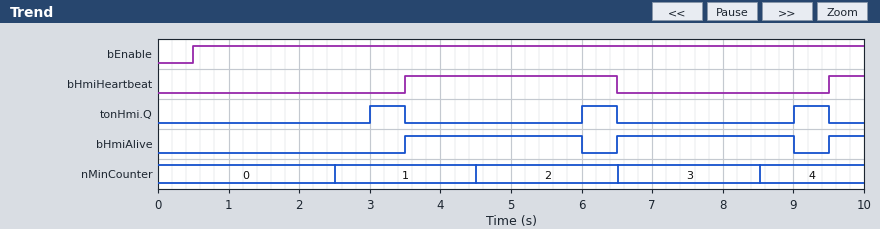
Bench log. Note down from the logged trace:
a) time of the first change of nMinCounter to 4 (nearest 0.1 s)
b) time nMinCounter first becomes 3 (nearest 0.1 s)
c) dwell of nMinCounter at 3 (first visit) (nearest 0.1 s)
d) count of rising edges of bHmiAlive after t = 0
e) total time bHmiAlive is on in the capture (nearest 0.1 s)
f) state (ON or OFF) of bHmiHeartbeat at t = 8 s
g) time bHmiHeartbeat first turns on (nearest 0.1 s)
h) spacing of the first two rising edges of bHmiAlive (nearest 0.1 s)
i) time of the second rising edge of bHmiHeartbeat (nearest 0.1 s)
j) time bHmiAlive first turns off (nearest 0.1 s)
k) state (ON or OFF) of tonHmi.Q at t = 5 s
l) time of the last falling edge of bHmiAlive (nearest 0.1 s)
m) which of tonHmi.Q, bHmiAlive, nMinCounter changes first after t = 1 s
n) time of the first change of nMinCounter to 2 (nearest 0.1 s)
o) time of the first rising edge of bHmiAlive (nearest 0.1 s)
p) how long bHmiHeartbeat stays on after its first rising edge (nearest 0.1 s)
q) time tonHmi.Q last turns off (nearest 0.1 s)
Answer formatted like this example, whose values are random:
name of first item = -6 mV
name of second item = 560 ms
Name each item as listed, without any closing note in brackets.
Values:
time of the first change of nMinCounter to 4 = 8.5 s
time nMinCounter first becomes 3 = 6.5 s
dwell of nMinCounter at 3 (first visit) = 2.0 s
count of rising edges of bHmiAlive after t = 0 = 3
total time bHmiAlive is on in the capture = 5.5 s
state (ON or OFF) of bHmiHeartbeat at t = 8 s = OFF
time bHmiHeartbeat first turns on = 3.5 s
spacing of the first two rising edges of bHmiAlive = 3.0 s
time of the second rising edge of bHmiHeartbeat = 9.5 s
time bHmiAlive first turns off = 6.0 s
state (ON or OFF) of tonHmi.Q at t = 5 s = OFF
time of the last falling edge of bHmiAlive = 9.0 s
which of tonHmi.Q, bHmiAlive, nMinCounter changes first after t = 1 s = nMinCounter
time of the first change of nMinCounter to 2 = 4.5 s
time of the first rising edge of bHmiAlive = 3.5 s
how long bHmiHeartbeat stays on after its first rising edge = 3.0 s
time tonHmi.Q last turns off = 9.5 s
